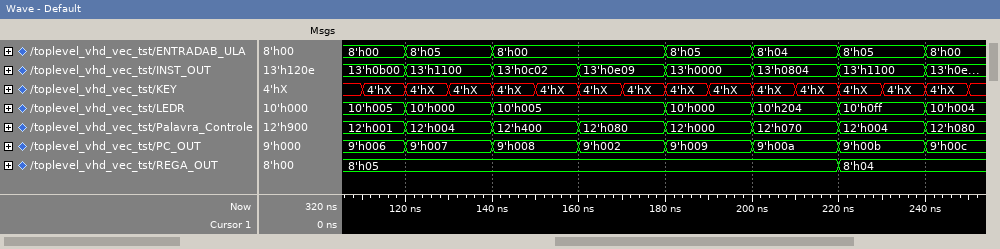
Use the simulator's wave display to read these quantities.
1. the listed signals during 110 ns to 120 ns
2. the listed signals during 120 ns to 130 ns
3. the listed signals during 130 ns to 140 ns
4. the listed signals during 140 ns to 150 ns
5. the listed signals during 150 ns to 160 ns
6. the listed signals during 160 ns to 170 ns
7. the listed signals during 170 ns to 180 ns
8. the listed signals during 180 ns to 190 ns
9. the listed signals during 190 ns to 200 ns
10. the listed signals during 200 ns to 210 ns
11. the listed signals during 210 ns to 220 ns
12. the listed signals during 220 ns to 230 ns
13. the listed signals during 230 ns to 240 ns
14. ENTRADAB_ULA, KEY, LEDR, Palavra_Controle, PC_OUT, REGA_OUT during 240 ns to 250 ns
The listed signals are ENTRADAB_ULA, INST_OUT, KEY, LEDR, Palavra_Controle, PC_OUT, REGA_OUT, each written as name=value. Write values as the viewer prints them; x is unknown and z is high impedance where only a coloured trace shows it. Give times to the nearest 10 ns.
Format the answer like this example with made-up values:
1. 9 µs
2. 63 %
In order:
1. ENTRADAB_ULA=8'h00, INST_OUT=13'h0b00, KEY=4'hX, LEDR=10'h005, Palavra_Controle=12'h001, PC_OUT=9'h006, REGA_OUT=8'h05
2. ENTRADAB_ULA=8'h05, INST_OUT=13'h1100, KEY=4'hX, LEDR=10'h000, Palavra_Controle=12'h004, PC_OUT=9'h007, REGA_OUT=8'h05
3. ENTRADAB_ULA=8'h05, INST_OUT=13'h1100, KEY=4'hX, LEDR=10'h000, Palavra_Controle=12'h004, PC_OUT=9'h007, REGA_OUT=8'h05
4. ENTRADAB_ULA=8'h00, INST_OUT=13'h0c02, KEY=4'hX, LEDR=10'h005, Palavra_Controle=12'h400, PC_OUT=9'h008, REGA_OUT=8'h05
5. ENTRADAB_ULA=8'h00, INST_OUT=13'h0c02, KEY=4'hX, LEDR=10'h005, Palavra_Controle=12'h400, PC_OUT=9'h008, REGA_OUT=8'h05
6. ENTRADAB_ULA=8'h00, INST_OUT=13'h0e09, KEY=4'hX, LEDR=10'h005, Palavra_Controle=12'h080, PC_OUT=9'h002, REGA_OUT=8'h05
7. ENTRADAB_ULA=8'h00, INST_OUT=13'h0e09, KEY=4'hX, LEDR=10'h005, Palavra_Controle=12'h080, PC_OUT=9'h002, REGA_OUT=8'h05
8. ENTRADAB_ULA=8'h05, INST_OUT=13'h0000, KEY=4'hX, LEDR=10'h000, Palavra_Controle=12'h000, PC_OUT=9'h009, REGA_OUT=8'h05
9. ENTRADAB_ULA=8'h05, INST_OUT=13'h0000, KEY=4'hX, LEDR=10'h000, Palavra_Controle=12'h000, PC_OUT=9'h009, REGA_OUT=8'h05
10. ENTRADAB_ULA=8'h04, INST_OUT=13'h0804, KEY=4'hX, LEDR=10'h204, Palavra_Controle=12'h070, PC_OUT=9'h00a, REGA_OUT=8'h05
11. ENTRADAB_ULA=8'h04, INST_OUT=13'h0804, KEY=4'hX, LEDR=10'h204, Palavra_Controle=12'h070, PC_OUT=9'h00a, REGA_OUT=8'h05
12. ENTRADAB_ULA=8'h05, INST_OUT=13'h1100, KEY=4'hX, LEDR=10'h0ff, Palavra_Controle=12'h004, PC_OUT=9'h00b, REGA_OUT=8'h04
13. ENTRADAB_ULA=8'h05, INST_OUT=13'h1100, KEY=4'hX, LEDR=10'h0ff, Palavra_Controle=12'h004, PC_OUT=9'h00b, REGA_OUT=8'h04
14. ENTRADAB_ULA=8'h00, KEY=4'hX, LEDR=10'h004, Palavra_Controle=12'h080, PC_OUT=9'h00c, REGA_OUT=8'h04
